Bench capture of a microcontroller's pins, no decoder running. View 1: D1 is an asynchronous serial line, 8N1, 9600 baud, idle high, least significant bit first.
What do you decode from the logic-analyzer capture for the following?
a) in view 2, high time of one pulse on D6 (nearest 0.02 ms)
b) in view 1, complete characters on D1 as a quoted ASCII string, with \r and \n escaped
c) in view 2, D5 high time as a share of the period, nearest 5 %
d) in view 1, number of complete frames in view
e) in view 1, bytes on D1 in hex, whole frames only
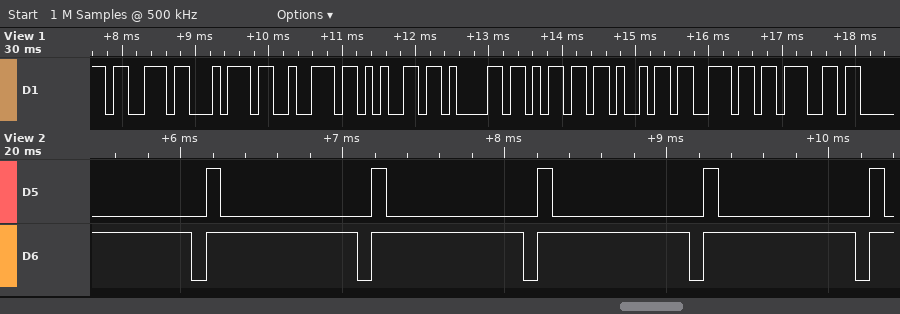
0.94 ms
"streaming"
10 %
9
73 74 72 65 61 6D 69 6E 67
